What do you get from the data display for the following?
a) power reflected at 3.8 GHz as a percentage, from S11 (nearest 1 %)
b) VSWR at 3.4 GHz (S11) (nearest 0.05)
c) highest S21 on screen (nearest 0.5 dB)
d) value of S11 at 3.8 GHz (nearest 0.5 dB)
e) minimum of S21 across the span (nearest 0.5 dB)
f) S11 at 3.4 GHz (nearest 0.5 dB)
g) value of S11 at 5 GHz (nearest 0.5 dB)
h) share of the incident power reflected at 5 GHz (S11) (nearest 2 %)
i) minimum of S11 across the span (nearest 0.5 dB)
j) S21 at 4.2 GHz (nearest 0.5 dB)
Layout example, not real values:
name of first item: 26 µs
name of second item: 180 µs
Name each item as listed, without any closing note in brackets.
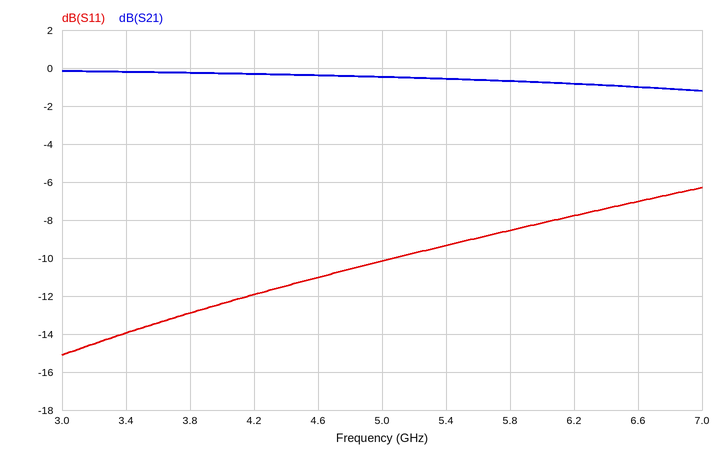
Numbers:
power reflected at 3.8 GHz as a percentage, from S11: 5 %
VSWR at 3.4 GHz (S11): 1.50
highest S21 on screen: 0.0 dB
value of S11 at 3.8 GHz: -13.0 dB
minimum of S21 across the span: -1.0 dB
S11 at 3.4 GHz: -14.0 dB
value of S11 at 5 GHz: -10.0 dB
share of the incident power reflected at 5 GHz (S11): 10 %
minimum of S11 across the span: -15.0 dB
S21 at 4.2 GHz: -0.5 dB
